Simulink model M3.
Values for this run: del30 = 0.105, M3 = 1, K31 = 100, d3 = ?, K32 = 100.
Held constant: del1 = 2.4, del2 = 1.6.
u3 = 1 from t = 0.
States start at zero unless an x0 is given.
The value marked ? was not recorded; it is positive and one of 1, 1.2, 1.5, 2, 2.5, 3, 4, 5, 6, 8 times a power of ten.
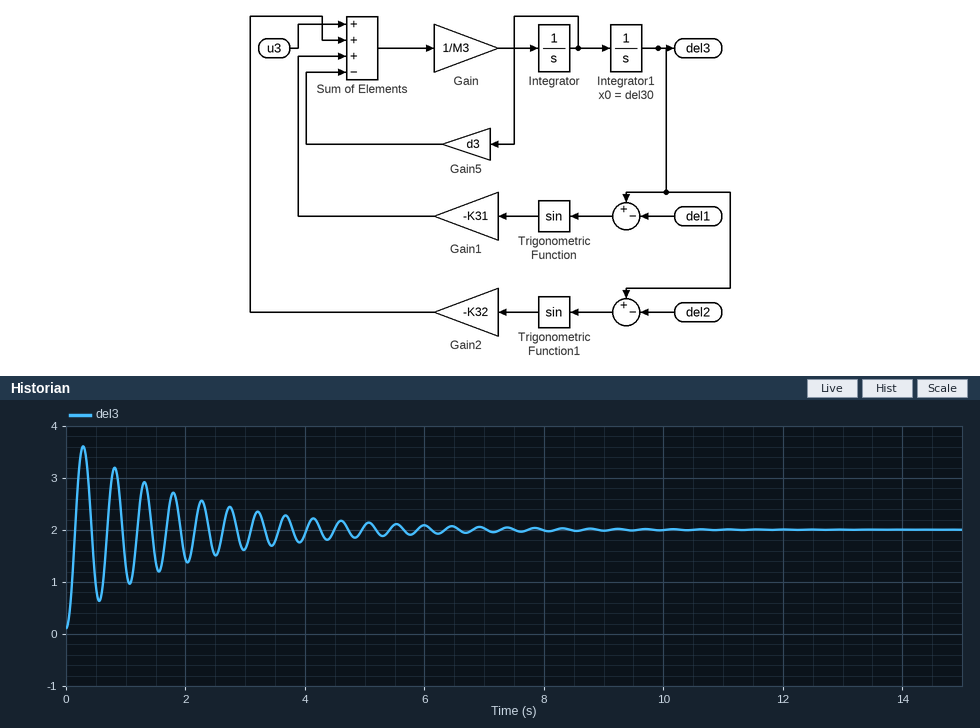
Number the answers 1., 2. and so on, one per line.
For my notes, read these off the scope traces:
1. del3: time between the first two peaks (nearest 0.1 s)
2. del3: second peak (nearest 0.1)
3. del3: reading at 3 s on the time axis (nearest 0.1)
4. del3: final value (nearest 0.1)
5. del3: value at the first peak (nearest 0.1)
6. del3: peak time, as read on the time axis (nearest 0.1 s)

1. 0.5 s
2. 3.2
3. 1.6
4. 2.0
5. 3.6
6. 0.3 s
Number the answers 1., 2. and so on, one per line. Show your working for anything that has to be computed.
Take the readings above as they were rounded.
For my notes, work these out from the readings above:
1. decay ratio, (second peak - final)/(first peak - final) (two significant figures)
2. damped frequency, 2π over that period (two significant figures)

1. (3.2 - 2) / (3.6 - 2) = 0.75
2. 2π / 0.5 = 13 rad/s
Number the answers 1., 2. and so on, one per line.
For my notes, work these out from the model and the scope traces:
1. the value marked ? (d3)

1. 1
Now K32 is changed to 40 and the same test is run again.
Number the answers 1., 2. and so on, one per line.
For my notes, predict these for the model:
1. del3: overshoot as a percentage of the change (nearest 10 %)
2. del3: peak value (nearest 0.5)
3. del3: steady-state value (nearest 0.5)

1. 80 %
2. 4.0
3. 2.0
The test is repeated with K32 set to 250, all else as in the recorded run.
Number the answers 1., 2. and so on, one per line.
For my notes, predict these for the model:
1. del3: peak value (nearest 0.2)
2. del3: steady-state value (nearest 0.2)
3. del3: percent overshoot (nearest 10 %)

1. 3.4
2. 1.8
3. 90 %
